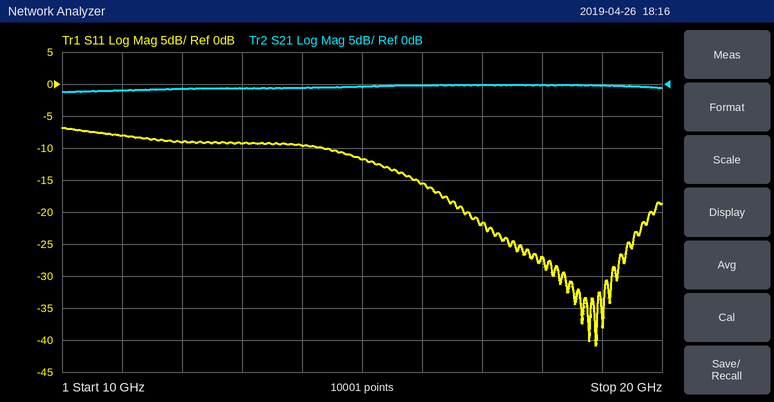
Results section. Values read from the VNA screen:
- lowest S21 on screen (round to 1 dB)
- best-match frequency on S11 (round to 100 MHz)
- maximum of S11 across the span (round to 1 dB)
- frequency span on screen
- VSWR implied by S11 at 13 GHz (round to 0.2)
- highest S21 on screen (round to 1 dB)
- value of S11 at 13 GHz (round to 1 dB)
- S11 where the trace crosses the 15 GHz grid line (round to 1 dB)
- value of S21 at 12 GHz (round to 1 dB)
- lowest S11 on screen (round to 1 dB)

-1 dB
18.9 GHz
-7 dB
10 GHz
2.0
0 dB
-9 dB
-12 dB
-1 dB
-41 dB
